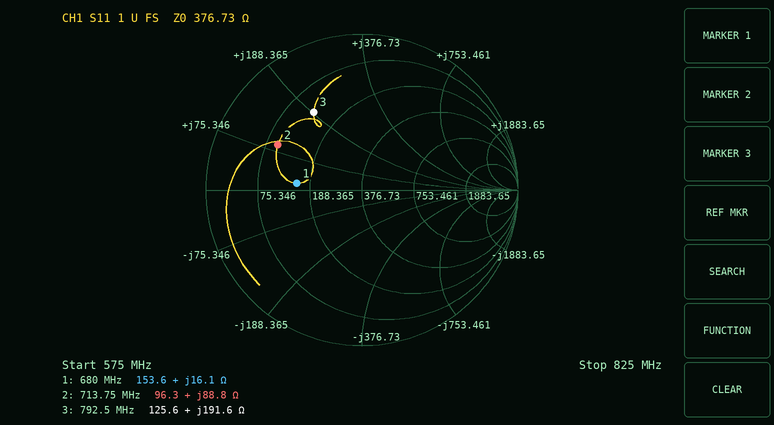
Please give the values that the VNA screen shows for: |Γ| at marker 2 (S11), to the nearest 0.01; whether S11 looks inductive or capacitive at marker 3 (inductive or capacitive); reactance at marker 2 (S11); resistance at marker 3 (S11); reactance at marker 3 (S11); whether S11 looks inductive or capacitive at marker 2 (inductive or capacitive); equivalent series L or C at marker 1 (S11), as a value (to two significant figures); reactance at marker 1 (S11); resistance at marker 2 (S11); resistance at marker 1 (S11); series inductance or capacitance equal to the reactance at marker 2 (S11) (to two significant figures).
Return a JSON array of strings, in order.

["0.61", "inductive", "+88.8 Ω", "125.6 Ω", "+191.6 Ω", "inductive", "3.8 nH", "+16.1 Ω", "96.3 Ω", "153.6 Ω", "20 nH"]
